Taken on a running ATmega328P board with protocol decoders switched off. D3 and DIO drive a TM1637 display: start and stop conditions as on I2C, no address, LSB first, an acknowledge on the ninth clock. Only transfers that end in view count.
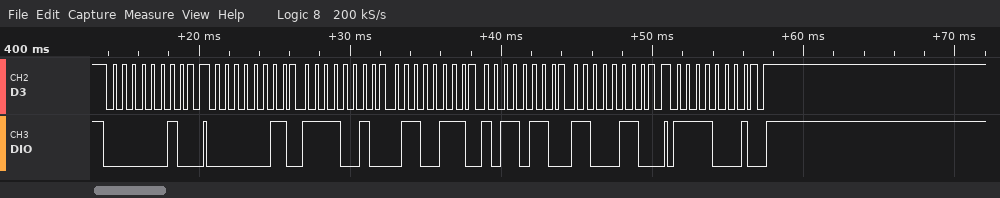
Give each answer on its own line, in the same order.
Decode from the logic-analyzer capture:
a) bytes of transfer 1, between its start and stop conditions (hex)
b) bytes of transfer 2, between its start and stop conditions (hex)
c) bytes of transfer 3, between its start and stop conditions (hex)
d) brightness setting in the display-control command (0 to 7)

40
C0 4F E6 6D 63
8F
7
